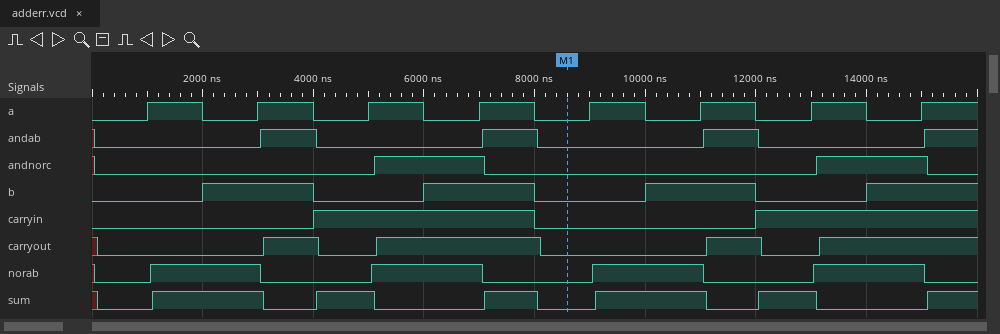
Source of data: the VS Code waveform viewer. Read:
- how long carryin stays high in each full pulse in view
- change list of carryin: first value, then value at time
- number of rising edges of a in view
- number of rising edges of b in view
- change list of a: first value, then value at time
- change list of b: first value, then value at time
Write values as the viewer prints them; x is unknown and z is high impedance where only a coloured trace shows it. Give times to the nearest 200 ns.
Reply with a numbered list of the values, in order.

1. 4000 ns
2. 0, 1 at 4000 ns, 0 at 8000 ns, 1 at 12000 ns
3. 8
4. 4
5. 0, 1 at 1000 ns, 0 at 2000 ns, 1 at 3000 ns, 0 at 4000 ns, 1 at 5000 ns, 0 at 6000 ns, 1 at 7000 ns, 0 at 8000 ns, 1 at 9000 ns, 0 at 10000 ns, 1 at 11000 ns, 0 at 12000 ns, 1 at 13000 ns, 0 at 14000 ns, 1 at 15000 ns
6. 0, 1 at 2000 ns, 0 at 4000 ns, 1 at 6000 ns, 0 at 8000 ns, 1 at 10000 ns, 0 at 12000 ns, 1 at 14000 ns
